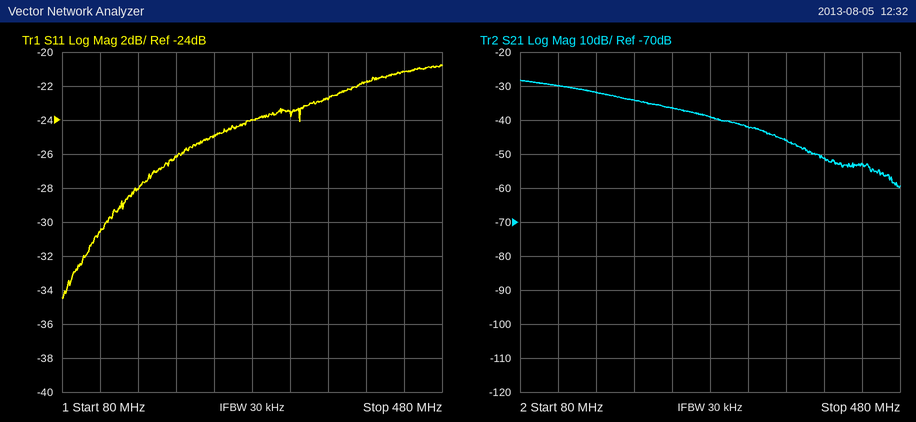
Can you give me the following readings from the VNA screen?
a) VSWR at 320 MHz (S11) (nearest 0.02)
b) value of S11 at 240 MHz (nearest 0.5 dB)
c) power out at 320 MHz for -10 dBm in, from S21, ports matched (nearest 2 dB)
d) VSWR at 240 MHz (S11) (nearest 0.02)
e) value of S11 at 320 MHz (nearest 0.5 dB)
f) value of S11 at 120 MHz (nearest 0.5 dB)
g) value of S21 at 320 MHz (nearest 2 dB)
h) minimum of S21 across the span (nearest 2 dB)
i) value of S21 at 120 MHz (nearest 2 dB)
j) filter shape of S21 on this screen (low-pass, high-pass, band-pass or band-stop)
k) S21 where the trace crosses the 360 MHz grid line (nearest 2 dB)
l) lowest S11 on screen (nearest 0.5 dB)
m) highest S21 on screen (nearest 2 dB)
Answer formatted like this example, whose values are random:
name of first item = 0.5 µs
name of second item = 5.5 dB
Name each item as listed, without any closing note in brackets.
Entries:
VSWR at 320 MHz (S11) = 1.14
value of S11 at 240 MHz = -25.0 dB
power out at 320 MHz for -10 dBm in, from S21, ports matched = -52 dBm
VSWR at 240 MHz (S11) = 1.12
value of S11 at 320 MHz = -23.5 dB
value of S11 at 120 MHz = -30.5 dB
value of S21 at 320 MHz = -42 dB
minimum of S21 across the span = -60 dB
value of S21 at 120 MHz = -30 dB
filter shape of S21 on this screen = low-pass
S21 where the trace crosses the 360 MHz grid line = -46 dB
lowest S11 on screen = -34.5 dB
highest S21 on screen = -28 dB
